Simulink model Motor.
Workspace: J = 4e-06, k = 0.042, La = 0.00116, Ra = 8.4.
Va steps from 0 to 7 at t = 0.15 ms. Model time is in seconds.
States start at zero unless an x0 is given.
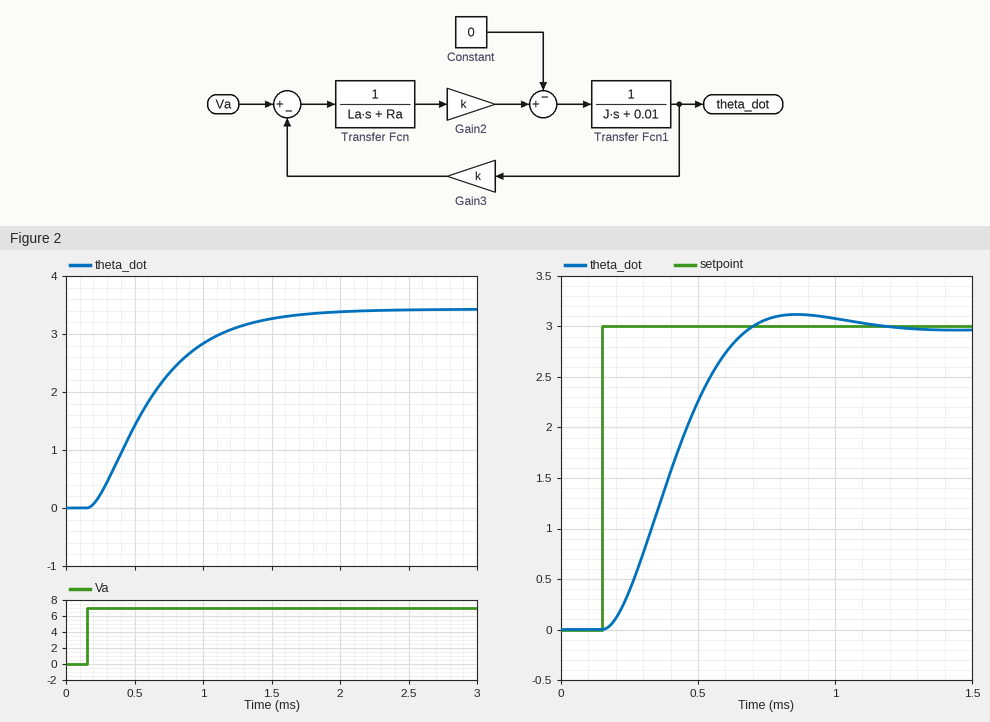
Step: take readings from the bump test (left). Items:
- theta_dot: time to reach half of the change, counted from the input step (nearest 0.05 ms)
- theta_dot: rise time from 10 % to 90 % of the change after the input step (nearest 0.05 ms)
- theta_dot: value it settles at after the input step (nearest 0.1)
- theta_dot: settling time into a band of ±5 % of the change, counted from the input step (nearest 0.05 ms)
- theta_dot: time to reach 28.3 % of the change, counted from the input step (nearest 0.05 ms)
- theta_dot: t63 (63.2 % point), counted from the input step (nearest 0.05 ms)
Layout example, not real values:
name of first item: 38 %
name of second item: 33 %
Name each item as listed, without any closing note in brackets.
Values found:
theta_dot: time to reach half of the change, counted from the input step: 0.40 ms
theta_dot: rise time from 10 % to 90 % of the change after the input step: 0.95 ms
theta_dot: value it settles at after the input step: 3.4
theta_dot: settling time into a band of ±5 % of the change, counted from the input step: 1.35 ms
theta_dot: time to reach 28.3 % of the change, counted from the input step: 0.25 ms
theta_dot: t63 (63.2 % point), counted from the input step: 0.55 ms
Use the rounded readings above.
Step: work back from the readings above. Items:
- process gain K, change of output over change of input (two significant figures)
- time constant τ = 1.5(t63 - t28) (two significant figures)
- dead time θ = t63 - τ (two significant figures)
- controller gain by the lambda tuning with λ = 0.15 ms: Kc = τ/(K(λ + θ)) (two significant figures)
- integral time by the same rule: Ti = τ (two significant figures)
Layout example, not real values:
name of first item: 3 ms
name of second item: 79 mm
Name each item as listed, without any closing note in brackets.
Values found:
process gain K, change of output over change of input: 0.49
time constant τ = 1.5(t63 - t28): 0.45 ms
dead time θ = t63 - τ: 0.10 ms
controller gain by the lambda tuning with λ = 0.15 ms: Kc = τ/(K(λ + θ)): 3.7
integral time by the same rule: Ti = τ: 0.45 ms
